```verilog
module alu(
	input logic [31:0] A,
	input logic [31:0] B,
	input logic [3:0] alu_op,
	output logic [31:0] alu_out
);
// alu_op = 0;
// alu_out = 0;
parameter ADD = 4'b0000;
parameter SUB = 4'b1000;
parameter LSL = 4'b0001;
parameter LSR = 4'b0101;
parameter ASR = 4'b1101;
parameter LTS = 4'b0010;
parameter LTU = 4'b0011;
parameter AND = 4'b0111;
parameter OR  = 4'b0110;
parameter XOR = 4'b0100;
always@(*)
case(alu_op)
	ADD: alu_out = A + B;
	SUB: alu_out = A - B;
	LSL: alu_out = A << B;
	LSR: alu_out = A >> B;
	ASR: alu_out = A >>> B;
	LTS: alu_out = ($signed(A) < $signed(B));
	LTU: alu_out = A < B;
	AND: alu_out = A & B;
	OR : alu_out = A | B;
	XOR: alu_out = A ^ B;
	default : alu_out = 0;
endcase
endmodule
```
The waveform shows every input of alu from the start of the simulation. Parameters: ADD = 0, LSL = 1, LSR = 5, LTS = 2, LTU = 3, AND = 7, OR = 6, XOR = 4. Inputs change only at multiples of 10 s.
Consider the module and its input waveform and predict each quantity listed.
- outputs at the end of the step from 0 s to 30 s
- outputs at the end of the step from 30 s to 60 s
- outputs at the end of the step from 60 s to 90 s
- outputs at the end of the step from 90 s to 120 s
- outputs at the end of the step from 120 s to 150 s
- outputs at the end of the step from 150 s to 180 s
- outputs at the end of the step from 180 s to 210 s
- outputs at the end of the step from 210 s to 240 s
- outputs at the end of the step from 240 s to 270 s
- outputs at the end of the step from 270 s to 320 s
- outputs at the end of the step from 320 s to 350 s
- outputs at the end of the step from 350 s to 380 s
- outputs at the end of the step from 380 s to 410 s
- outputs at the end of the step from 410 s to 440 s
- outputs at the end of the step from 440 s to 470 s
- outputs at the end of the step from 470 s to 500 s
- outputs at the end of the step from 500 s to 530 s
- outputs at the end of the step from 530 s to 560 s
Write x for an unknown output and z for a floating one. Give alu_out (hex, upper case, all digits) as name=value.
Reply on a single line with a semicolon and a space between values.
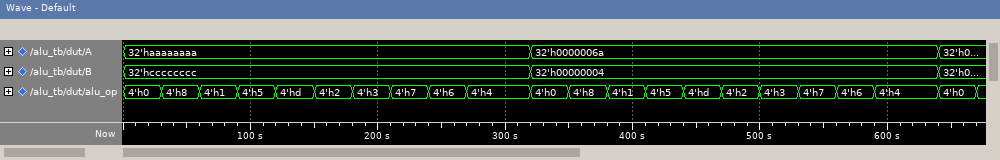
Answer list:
alu_out=77777776; alu_out=DDDDDDDE; alu_out=00000000; alu_out=00000000; alu_out=00000000; alu_out=00000001; alu_out=00000001; alu_out=88888888; alu_out=EEEEEEEE; alu_out=66666666; alu_out=0000006E; alu_out=00000066; alu_out=000006A0; alu_out=00000006; alu_out=00000006; alu_out=00000000; alu_out=00000000; alu_out=00000000
